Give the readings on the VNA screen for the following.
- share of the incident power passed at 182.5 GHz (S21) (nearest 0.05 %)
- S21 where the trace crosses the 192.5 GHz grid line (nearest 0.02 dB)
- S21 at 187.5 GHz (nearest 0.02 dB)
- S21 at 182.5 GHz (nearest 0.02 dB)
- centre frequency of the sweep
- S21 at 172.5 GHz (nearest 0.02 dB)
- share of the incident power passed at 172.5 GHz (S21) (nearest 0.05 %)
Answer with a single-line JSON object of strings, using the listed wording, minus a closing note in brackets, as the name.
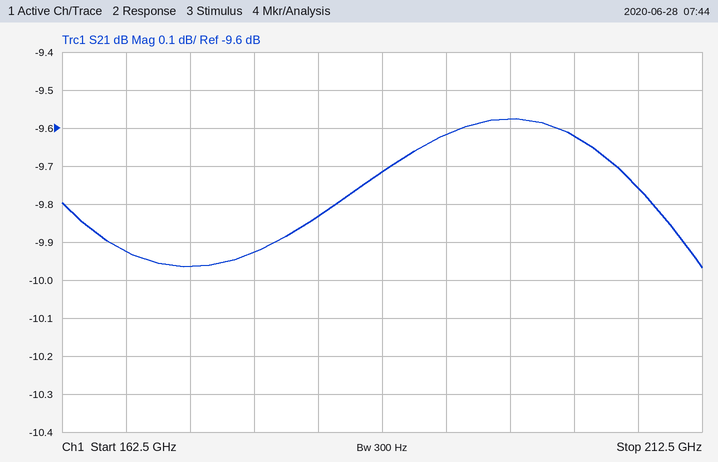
{"share of the incident power passed at 182.5 GHz (S21)": "10.40 %", "S21 where the trace crosses the 192.5 GHz grid line": "-9.62 dB", "S21 at 187.5 GHz": "-9.72 dB", "S21 at 182.5 GHz": "-9.84 dB", "centre frequency of the sweep": "187.5 GHz", "S21 at 172.5 GHz": "-9.96 dB", "share of the incident power passed at 172.5 GHz (S21)": "10.10 %"}
